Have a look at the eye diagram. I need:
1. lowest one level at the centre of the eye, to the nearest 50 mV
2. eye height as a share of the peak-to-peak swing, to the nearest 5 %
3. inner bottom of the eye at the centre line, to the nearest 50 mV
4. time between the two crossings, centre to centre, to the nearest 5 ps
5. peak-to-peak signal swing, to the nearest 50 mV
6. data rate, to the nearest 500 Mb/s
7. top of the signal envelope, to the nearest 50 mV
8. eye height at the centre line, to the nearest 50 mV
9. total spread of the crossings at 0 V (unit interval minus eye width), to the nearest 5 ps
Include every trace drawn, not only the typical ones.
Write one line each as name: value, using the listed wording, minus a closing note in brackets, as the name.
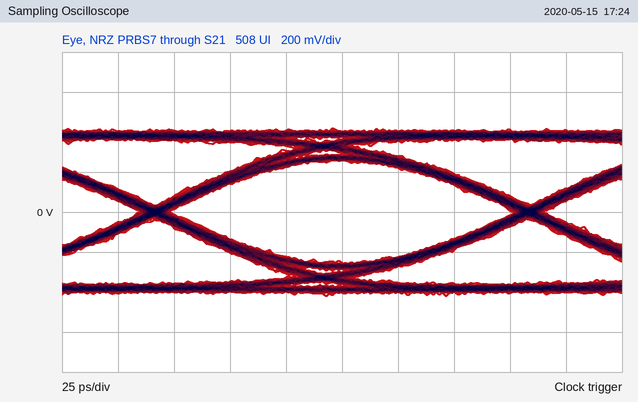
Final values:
lowest one level at the centre of the eye, to the nearest 50 mV: 250 mV
eye height as a share of the peak-to-peak swing, to the nearest 5 %: 60 %
inner bottom of the eye at the centre line, to the nearest 50 mV: -250 mV
time between the two crossings, centre to centre, to the nearest 5 ps: 165 ps
peak-to-peak signal swing, to the nearest 50 mV: 850 mV
data rate, to the nearest 500 Mb/s: 6.0 Gb/s
top of the signal envelope, to the nearest 50 mV: 400 mV
eye height at the centre line, to the nearest 50 mV: 500 mV
total spread of the crossings at 0 V (unit interval minus eye width), to the nearest 5 ps: 15 ps
